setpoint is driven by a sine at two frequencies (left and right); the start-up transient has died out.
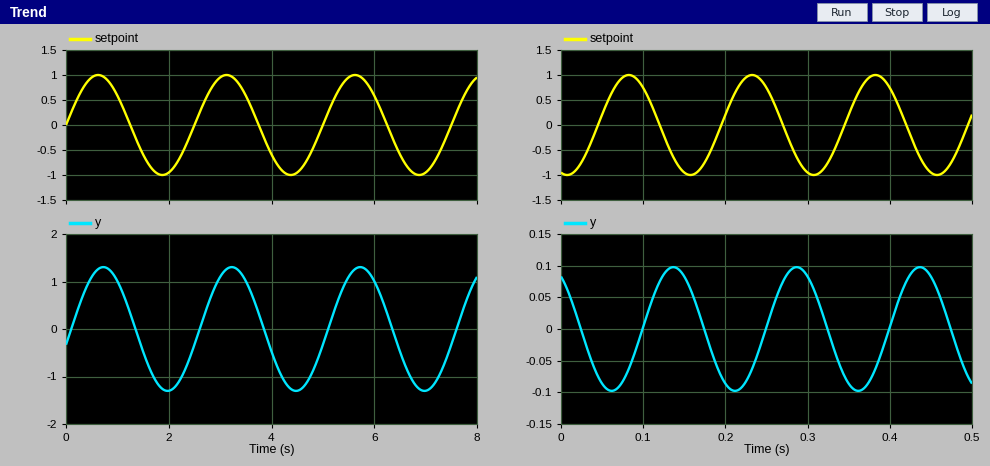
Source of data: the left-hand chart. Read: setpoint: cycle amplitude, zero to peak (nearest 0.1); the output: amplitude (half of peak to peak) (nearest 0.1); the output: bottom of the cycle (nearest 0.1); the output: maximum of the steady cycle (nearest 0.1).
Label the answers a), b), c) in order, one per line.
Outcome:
a) 1.0
b) 1.3
c) -1.3
d) 1.3
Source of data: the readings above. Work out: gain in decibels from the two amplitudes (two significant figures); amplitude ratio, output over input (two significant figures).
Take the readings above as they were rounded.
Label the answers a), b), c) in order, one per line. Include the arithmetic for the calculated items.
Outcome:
a) 20 log10(1.3 / 1) = 2.3 dB
b) 1.3 / 1 = 1.3
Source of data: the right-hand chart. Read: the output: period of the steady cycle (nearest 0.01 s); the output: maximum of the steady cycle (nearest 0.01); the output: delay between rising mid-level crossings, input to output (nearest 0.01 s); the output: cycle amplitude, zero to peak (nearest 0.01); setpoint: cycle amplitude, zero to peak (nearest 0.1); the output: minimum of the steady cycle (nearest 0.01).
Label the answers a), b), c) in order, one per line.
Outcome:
a) 0.15 s
b) 0.10
c) 0.05 s
d) 0.10
e) 1.0
f) -0.10
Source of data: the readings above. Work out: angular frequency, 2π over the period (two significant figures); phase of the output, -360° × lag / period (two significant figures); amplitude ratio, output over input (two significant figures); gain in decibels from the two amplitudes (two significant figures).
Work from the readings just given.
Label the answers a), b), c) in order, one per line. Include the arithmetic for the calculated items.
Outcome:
a) 2π / 0.15 = 42 rad/s
b) -360 × 0.05 / 0.15 = -120°
c) 0.1 / 1 = 0.10
d) 20 log10(0.1 / 1) = -20 dB
